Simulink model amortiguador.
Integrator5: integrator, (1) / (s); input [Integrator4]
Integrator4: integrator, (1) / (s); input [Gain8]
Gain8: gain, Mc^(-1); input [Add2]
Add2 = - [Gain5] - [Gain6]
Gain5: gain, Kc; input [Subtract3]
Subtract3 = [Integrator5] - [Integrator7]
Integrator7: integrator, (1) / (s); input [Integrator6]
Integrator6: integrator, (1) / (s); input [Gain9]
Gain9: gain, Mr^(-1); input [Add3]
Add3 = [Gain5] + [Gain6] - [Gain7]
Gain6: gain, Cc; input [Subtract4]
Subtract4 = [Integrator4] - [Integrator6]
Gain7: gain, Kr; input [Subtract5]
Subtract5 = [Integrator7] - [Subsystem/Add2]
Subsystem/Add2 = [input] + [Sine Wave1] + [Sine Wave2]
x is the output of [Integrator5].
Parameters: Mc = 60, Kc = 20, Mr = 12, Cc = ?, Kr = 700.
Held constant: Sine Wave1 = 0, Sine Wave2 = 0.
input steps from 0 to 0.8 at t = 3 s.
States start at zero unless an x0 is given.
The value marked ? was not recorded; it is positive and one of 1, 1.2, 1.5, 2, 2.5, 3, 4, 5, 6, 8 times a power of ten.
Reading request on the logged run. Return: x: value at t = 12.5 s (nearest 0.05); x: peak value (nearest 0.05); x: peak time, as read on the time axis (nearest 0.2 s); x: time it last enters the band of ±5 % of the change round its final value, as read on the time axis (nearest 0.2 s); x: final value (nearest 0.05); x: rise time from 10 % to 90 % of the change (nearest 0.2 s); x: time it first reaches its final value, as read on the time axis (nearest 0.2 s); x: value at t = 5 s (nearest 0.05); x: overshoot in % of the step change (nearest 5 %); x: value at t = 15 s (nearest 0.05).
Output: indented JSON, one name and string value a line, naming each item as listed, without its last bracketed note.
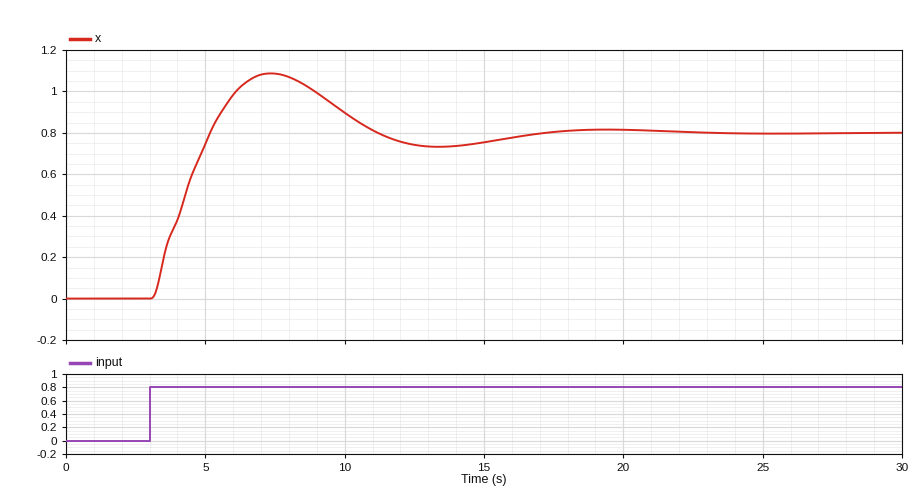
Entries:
{
  "x: value at t = 12.5 s": "0.75",
  "x: peak value": "1.10",
  "x: peak time, as read on the time axis": "7.4 s",
  "x: time it last enters the band of ±5 % of the change round its final value, as read on the time axis": "15.2 s",
  "x: final value": "0.80",
  "x: rise time from 10 % to 90 % of the change": "1.6 s",
  "x: time it first reaches its final value, as read on the time axis": "5.2 s",
  "x: value at t = 5 s": "0.75",
  "x: overshoot in % of the step change": "35 %",
  "x: value at t = 15 s": "0.75"
}
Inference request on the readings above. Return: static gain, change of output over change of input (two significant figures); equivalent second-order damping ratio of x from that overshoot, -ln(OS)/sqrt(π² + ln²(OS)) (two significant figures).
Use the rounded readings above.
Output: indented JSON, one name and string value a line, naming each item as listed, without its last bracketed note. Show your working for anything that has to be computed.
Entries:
{
  "static gain, change of output over change of input": "(0.8 - 0) / (0.8 - 0) = 1.0",
  "equivalent second-order damping ratio of x from that overshoot, -ln(OS)/sqrt(π² + ln²(OS))": "ln(0.35) = -1.050; 1.050 / sqrt(9.870 + 1.102) = 0.32"
}
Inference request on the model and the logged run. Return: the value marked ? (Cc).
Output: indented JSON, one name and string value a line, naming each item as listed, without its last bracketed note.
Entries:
{
  "the value marked ?": "30"
}
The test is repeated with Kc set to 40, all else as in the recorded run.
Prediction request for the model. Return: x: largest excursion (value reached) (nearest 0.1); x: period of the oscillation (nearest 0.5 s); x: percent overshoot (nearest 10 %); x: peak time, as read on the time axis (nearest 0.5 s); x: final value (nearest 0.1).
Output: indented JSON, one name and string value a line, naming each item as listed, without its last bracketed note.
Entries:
{
  "x: largest excursion (value reached)": "1.2",
  "x: period of the oscillation": "8.0 s",
  "x: percent overshoot": "50 %",
  "x: peak time, as read on the time axis": "6.5 s",
  "x: final value": "0.8"
}
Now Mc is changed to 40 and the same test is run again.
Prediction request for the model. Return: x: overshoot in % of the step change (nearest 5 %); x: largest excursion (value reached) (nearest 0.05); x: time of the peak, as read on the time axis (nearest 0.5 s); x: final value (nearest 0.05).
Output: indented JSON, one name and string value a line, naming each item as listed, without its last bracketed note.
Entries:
{
  "x: overshoot in % of the step change": "30 %",
  "x: largest excursion (value reached)": "1.05",
  "x: time of the peak, as read on the time axis": "6.5 s",
  "x: final value": "0.80"
}
